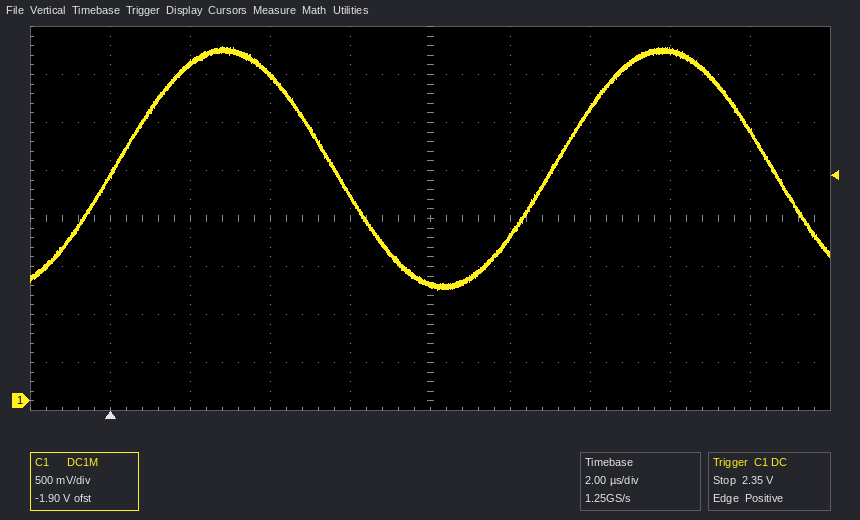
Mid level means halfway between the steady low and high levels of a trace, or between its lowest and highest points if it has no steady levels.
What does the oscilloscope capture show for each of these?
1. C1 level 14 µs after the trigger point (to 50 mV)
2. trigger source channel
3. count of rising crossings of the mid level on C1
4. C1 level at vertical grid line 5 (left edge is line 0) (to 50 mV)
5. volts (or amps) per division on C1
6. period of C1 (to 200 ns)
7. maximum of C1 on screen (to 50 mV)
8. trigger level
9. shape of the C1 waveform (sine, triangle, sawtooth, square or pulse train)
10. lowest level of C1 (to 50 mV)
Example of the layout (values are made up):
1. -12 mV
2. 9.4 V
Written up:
1. 3.65 V
2. C1
3. 2
4. 1.20 V
5. 500 mV
6. 11.0 µs
7. 3.70 V
8. 2.35 V
9. sine
10. 1.15 V
